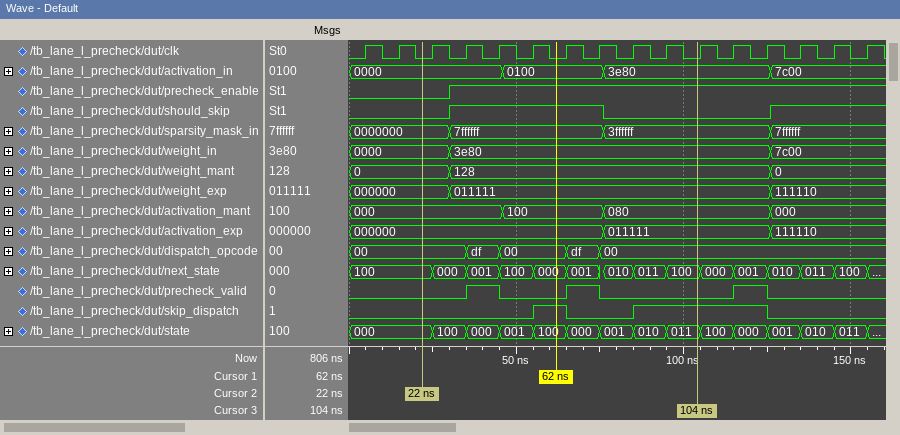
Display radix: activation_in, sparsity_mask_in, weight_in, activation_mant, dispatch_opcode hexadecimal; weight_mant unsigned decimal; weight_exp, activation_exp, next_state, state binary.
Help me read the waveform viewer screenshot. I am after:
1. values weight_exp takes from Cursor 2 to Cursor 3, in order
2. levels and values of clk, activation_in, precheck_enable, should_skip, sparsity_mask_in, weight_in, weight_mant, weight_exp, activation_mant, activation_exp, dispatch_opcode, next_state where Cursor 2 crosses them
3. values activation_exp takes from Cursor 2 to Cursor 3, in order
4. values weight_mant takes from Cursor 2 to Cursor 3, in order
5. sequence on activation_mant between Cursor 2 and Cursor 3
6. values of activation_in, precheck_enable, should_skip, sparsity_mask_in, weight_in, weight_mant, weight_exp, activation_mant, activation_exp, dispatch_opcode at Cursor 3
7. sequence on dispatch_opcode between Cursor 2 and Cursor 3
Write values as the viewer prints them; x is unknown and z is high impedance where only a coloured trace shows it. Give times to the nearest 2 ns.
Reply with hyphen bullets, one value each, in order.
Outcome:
- 000000, 011111
- clk=0, activation_in=0000, precheck_enable=0, should_skip=0, sparsity_mask_in=0000000, weight_in=0000, weight_mant=0, weight_exp=000000, activation_mant=000, activation_exp=000000, dispatch_opcode=00, next_state=100
- 000000, 011111
- 0, 128
- 000, 100, 080
- activation_in=3e80, precheck_enable=1, should_skip=0, sparsity_mask_in=3ffffff, weight_in=3e80, weight_mant=128, weight_exp=011111, activation_mant=080, activation_exp=011111, dispatch_opcode=00
- 00, df, 00, df, 00
